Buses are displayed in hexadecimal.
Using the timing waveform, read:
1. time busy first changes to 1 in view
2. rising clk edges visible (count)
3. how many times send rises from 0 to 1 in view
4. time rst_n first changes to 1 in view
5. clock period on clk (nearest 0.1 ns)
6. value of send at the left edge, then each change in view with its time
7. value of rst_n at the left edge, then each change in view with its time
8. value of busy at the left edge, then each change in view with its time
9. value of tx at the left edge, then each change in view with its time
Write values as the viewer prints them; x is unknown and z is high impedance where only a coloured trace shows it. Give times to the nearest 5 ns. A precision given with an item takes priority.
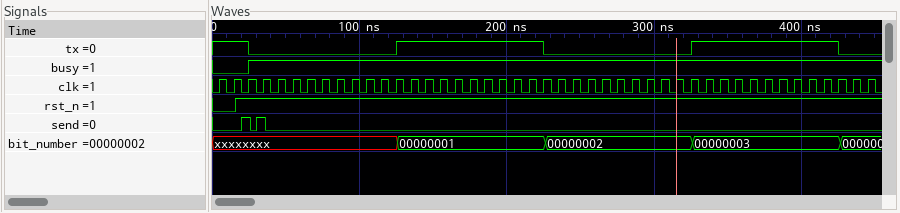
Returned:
25 ns
45
2
15 ns
10 ns
0, 1 at 20 ns, 0 at 25 ns, 1 at 30 ns, 0 at 35 ns
0, 1 at 15 ns
0, 1 at 25 ns
1, 0 at 25 ns, 1 at 125 ns, 0 at 225 ns, 1 at 325 ns, 0 at 425 ns
